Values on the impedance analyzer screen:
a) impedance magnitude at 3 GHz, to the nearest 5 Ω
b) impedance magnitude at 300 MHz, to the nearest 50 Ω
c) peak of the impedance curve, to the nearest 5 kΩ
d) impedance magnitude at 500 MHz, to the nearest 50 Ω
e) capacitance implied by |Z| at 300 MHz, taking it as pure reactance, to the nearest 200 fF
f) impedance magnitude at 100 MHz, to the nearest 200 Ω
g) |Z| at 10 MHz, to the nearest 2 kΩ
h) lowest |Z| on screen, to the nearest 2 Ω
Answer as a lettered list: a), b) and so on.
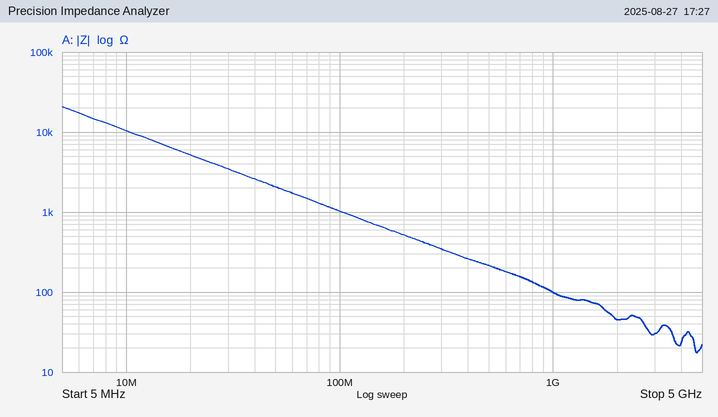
a) 30 Ω
b) 350 Ω
c) 20 kΩ
d) 200 Ω
e) 1.6 pF
f) 1.0 kΩ
g) 10 kΩ
h) 18 Ω
